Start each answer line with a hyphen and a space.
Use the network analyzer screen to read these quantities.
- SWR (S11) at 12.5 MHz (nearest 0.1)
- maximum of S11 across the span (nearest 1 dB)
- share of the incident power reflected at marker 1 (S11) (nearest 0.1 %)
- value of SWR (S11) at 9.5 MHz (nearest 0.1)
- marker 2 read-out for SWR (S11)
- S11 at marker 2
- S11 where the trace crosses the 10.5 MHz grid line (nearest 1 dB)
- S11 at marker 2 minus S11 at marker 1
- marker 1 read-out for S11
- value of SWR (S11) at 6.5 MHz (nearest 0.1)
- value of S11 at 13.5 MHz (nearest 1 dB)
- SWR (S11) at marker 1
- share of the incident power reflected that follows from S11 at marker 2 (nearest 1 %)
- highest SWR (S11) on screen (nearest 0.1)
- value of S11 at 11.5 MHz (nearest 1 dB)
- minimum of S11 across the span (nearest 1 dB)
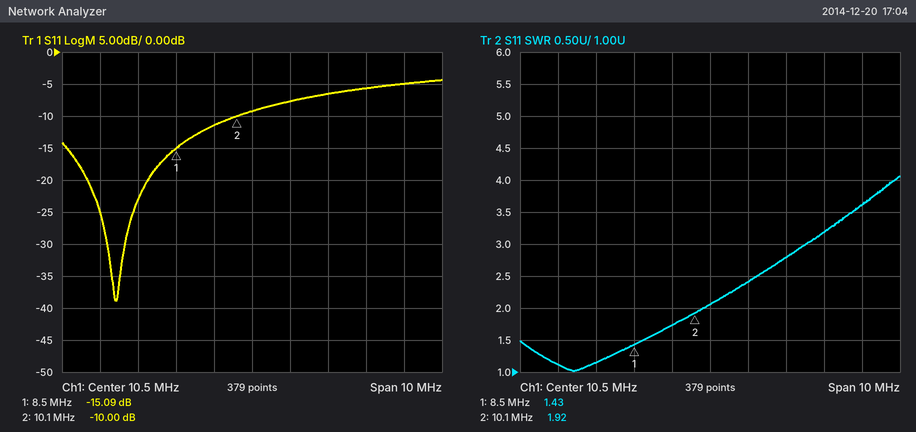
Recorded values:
- 2.8
- -4 dB
- 3.1 %
- 1.7
- 1.92
- -10.00 dB
- -9 dB
- 5.09 dB
- -15.09 dB
- 1.1
- -6 dB
- 1.43
- 10 %
- 4.1
- -8 dB
- -39 dB
